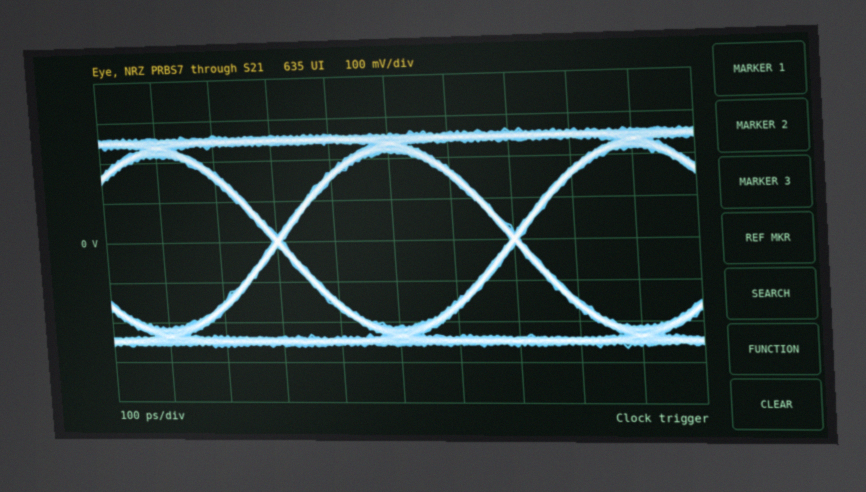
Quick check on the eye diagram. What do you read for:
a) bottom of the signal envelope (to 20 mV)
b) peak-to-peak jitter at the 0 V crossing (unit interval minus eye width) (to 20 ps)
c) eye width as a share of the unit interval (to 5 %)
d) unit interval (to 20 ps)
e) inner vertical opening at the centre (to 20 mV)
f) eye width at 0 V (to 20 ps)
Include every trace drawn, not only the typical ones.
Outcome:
-260 mV
20 ps
95 %
400 ps
420 mV
380 ps
